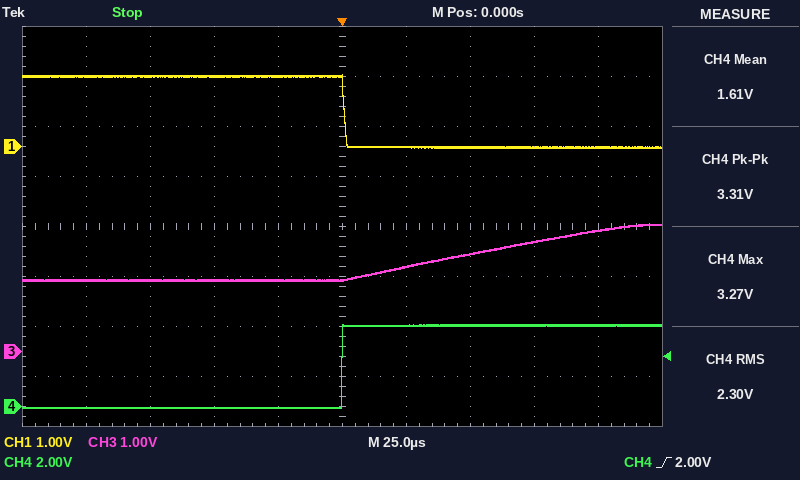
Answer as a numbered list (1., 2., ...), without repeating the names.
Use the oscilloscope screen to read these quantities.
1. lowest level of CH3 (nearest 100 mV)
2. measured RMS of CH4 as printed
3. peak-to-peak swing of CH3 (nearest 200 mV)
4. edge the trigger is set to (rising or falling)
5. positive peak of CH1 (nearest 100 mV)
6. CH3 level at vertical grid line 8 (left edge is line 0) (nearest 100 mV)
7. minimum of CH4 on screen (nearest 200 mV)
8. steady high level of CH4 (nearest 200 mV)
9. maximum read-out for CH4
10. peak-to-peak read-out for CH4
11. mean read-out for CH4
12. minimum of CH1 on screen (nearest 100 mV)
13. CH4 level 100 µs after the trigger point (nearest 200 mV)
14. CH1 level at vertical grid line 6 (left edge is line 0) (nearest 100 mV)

1. 1.4 V
2. 2.30 V
3. 1.2 V
4. rising
5. 1.4 V
6. 2.2 V
7. 0.0 V
8. 3.2 V
9. 3.27 V
10. 3.31 V
11. 1.61 V
12. 0.0 V
13. 3.2 V
14. 0.0 V
